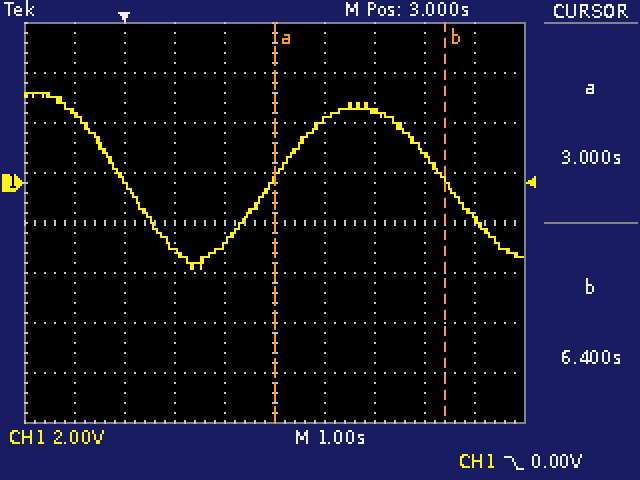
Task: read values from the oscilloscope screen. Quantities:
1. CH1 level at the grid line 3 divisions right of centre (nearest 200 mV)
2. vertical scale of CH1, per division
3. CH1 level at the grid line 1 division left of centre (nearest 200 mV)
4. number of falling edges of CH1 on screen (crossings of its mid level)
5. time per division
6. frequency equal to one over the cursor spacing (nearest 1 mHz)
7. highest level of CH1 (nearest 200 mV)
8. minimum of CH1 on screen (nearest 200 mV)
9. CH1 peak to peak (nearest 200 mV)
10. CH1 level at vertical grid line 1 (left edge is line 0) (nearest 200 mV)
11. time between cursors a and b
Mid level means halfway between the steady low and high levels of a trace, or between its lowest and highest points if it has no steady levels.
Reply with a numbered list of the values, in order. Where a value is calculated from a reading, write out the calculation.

1. 1.2 V
2. 2 V
3. -2.4 V
4. 2
5. 1 s
6. 1 / 3.4 s ≈ 294 mHz
7. 3.6 V
8. -3.4 V
9. 3.6 V − (-3.4 V) = 7.0 V
10. 2.8 V
11. 6.4 s − (3 s) = 3.4 s
